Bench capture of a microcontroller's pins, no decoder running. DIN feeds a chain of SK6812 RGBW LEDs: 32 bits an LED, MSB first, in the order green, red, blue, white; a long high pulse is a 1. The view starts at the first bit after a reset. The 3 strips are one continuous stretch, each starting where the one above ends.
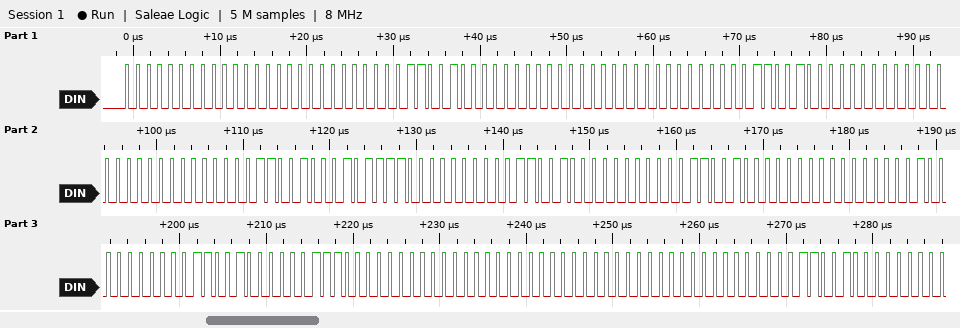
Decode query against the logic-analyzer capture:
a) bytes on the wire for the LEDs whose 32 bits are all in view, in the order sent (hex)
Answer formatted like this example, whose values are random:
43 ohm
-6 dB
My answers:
00 00 00 32 00 00 00 32 00 00 00 32 2F 00 32 00 32 00 01 00 32 07 00 00 00 00 00 32
